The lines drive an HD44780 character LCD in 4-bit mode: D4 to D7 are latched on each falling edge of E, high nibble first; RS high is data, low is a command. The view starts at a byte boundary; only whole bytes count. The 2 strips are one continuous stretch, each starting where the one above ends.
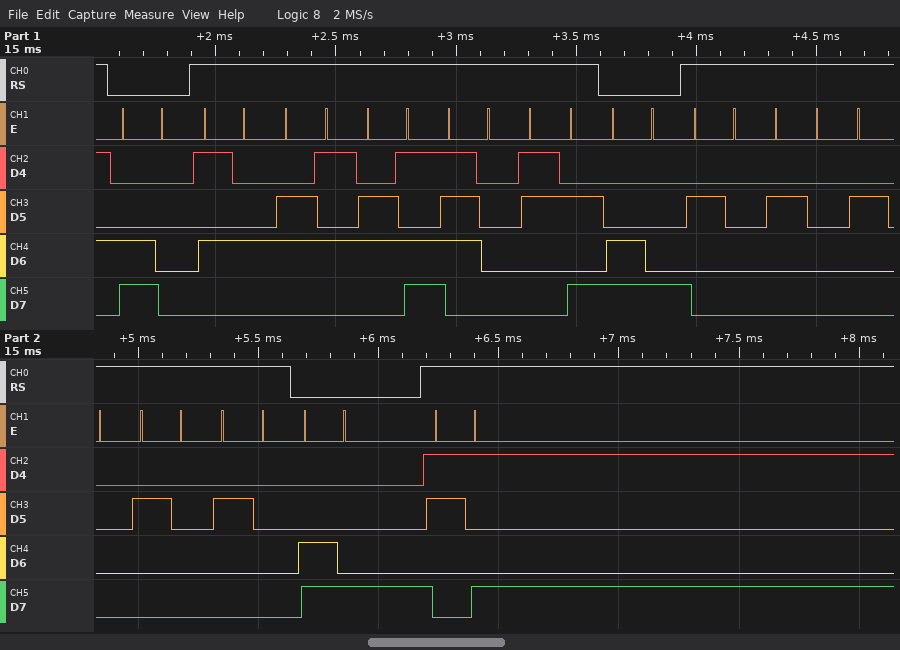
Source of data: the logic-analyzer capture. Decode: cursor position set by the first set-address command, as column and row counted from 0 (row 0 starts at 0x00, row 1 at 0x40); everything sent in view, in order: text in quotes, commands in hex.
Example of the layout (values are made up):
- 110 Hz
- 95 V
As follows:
- column 0, row 1
- 0xC0 "Temp:" 0xC8 "     " 0xC8 "9"
